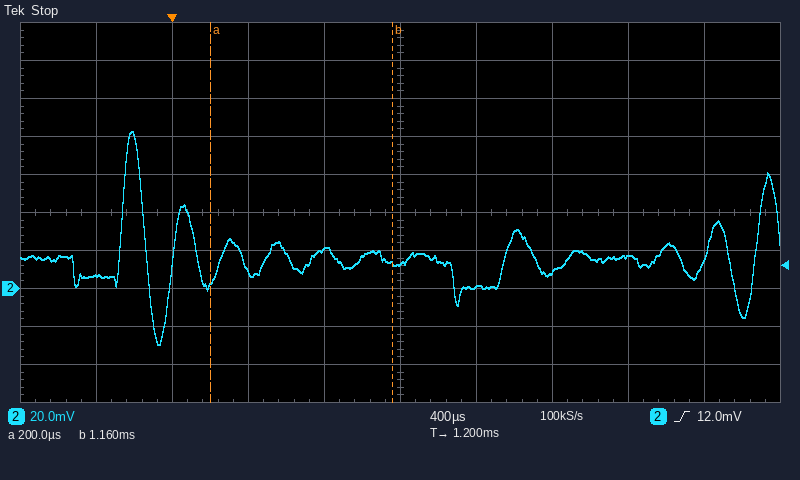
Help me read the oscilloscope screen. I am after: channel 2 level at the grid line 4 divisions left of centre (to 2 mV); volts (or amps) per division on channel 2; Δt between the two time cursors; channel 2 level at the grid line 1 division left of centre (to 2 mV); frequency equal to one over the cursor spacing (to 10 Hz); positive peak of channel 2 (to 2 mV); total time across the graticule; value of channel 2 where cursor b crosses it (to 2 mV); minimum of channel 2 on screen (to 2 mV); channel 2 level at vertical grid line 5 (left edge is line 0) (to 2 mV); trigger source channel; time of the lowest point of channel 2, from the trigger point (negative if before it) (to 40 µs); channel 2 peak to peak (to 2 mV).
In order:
6 mV
20 mV
960 µs
20 mV
1.04 kHz
82 mV
4 ms
14 mV
-30 mV
14 mV
channel 2
-80 µs
112 mV
